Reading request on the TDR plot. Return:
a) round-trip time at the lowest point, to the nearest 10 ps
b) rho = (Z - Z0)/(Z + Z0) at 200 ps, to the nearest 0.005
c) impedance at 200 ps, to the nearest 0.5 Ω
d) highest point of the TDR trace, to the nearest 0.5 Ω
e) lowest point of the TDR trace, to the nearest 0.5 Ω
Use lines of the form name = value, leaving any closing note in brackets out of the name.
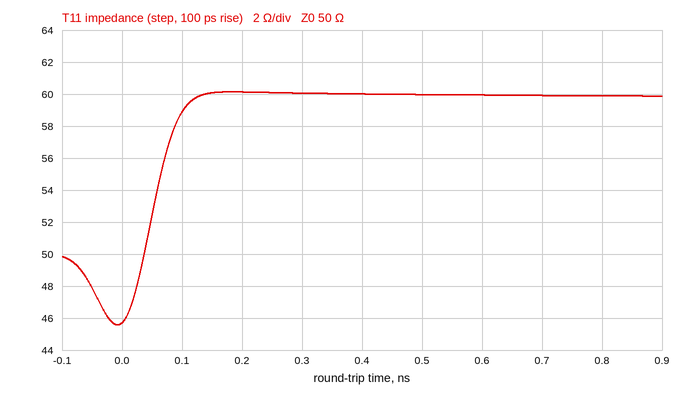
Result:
round-trip time at the lowest point, to the nearest 10 ps = -10 ps
rho = (Z - Z0)/(Z + Z0) at 200 ps, to the nearest 0.005 = +0.090
impedance at 200 ps, to the nearest 0.5 Ω = 60.0 Ω
highest point of the TDR trace, to the nearest 0.5 Ω = 60.0 Ω
lowest point of the TDR trace, to the nearest 0.5 Ω = 45.5 Ω
